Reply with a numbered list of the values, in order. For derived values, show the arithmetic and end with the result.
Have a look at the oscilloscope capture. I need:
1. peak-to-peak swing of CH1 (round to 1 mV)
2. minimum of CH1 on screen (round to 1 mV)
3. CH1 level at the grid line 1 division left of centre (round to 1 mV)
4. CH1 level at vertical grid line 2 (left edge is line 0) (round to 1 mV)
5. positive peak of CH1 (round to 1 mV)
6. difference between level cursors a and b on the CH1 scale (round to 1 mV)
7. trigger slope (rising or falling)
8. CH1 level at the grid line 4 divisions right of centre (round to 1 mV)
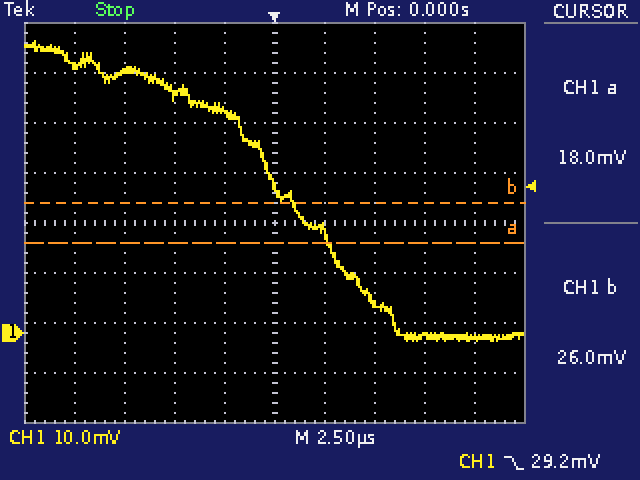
1. 58 mV − (-2 mV) = 60 mV
2. -2 mV
3. 44 mV
4. 52 mV
5. 58 mV
6. 8 mV
7. falling
8. -1 mV
